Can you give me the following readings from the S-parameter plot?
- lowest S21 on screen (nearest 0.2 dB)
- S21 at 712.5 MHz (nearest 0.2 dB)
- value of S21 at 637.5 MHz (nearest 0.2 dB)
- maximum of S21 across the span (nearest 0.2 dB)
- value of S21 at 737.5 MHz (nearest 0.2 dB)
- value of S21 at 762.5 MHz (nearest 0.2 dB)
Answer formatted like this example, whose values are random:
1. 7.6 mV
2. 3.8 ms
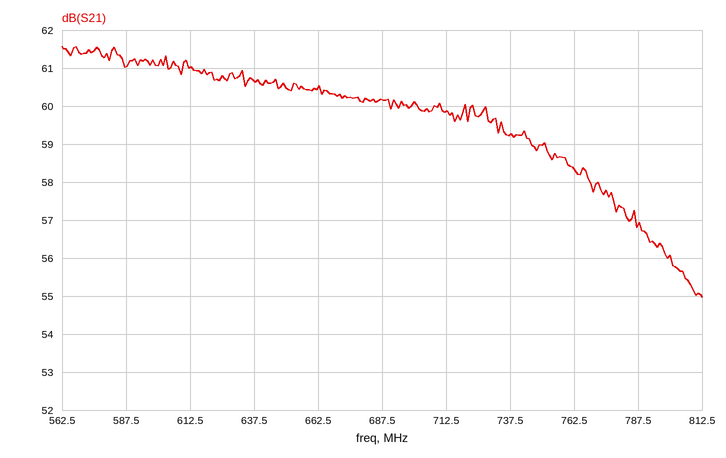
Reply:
1. 55.0 dB
2. 59.8 dB
3. 60.6 dB
4. 61.6 dB
5. 59.2 dB
6. 58.4 dB
